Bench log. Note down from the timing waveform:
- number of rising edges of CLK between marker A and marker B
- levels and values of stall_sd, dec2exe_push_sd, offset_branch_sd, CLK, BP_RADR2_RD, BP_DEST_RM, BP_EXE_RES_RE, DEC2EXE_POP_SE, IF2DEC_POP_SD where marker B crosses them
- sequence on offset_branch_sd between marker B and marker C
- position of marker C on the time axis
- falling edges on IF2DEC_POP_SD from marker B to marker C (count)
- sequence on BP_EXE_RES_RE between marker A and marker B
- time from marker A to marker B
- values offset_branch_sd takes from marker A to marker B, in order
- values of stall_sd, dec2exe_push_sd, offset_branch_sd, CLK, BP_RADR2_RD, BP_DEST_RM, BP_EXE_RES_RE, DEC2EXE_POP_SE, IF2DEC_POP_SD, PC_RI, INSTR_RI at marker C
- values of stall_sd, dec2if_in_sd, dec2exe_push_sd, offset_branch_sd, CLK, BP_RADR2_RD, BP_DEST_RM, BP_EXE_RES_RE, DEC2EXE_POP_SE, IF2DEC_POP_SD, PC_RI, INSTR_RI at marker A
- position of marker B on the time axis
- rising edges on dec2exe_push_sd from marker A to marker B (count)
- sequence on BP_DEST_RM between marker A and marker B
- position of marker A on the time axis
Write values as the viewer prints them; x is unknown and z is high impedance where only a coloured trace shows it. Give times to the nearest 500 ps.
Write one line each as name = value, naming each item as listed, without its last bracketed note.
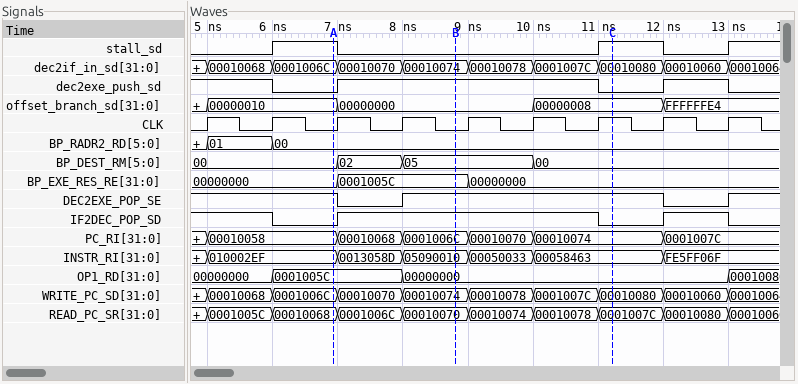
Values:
number of rising edges of CLK between marker A and marker B = 2
levels and values of stall_sd, dec2exe_push_sd, offset_branch_sd, CLK, BP_RADR2_RD, BP_DEST_RM, BP_EXE_RES_RE, DEC2EXE_POP_SE, IF2DEC_POP_SD where marker B crosses them = stall_sd=0, dec2exe_push_sd=1, offset_branch_sd=00000000, CLK=0, BP_RADR2_RD=00, BP_DEST_RM=05, BP_EXE_RES_RE=0001005C, DEC2EXE_POP_SE=1, IF2DEC_POP_SD=1
sequence on offset_branch_sd between marker B and marker C = 00000000, 00000008
position of marker C on the time axis = 11000 ps
falling edges on IF2DEC_POP_SD from marker B to marker C = 1
sequence on BP_EXE_RES_RE between marker A and marker B = 00000000, 0001005C
time from marker A to marker B = 2000 ps
values offset_branch_sd takes from marker A to marker B, in order = 00000010, 00000000
values of stall_sd, dec2exe_push_sd, offset_branch_sd, CLK, BP_RADR2_RD, BP_DEST_RM, BP_EXE_RES_RE, DEC2EXE_POP_SE, IF2DEC_POP_SD, PC_RI, INSTR_RI at marker C = stall_sd=1, dec2exe_push_sd=0, offset_branch_sd=00000008, CLK=1, BP_RADR2_RD=00, BP_DEST_RM=00, BP_EXE_RES_RE=00000000, DEC2EXE_POP_SE=1, IF2DEC_POP_SD=0, PC_RI=00010074, INSTR_RI=00058463
values of stall_sd, dec2if_in_sd, dec2exe_push_sd, offset_branch_sd, CLK, BP_RADR2_RD, BP_DEST_RM, BP_EXE_RES_RE, DEC2EXE_POP_SE, IF2DEC_POP_SD, PC_RI, INSTR_RI at marker A = stall_sd=1, dec2if_in_sd=0001006C, dec2exe_push_sd=0, offset_branch_sd=00000010, CLK=0, BP_RADR2_RD=00, BP_DEST_RM=00, BP_EXE_RES_RE=00000000, DEC2EXE_POP_SE=1, IF2DEC_POP_SD=0, PC_RI=00010058, INSTR_RI=010002EF
position of marker B on the time axis = 9000 ps
rising edges on dec2exe_push_sd from marker A to marker B = 1
sequence on BP_DEST_RM between marker A and marker B = 00, 02, 05
position of marker A on the time axis = 7000 ps
